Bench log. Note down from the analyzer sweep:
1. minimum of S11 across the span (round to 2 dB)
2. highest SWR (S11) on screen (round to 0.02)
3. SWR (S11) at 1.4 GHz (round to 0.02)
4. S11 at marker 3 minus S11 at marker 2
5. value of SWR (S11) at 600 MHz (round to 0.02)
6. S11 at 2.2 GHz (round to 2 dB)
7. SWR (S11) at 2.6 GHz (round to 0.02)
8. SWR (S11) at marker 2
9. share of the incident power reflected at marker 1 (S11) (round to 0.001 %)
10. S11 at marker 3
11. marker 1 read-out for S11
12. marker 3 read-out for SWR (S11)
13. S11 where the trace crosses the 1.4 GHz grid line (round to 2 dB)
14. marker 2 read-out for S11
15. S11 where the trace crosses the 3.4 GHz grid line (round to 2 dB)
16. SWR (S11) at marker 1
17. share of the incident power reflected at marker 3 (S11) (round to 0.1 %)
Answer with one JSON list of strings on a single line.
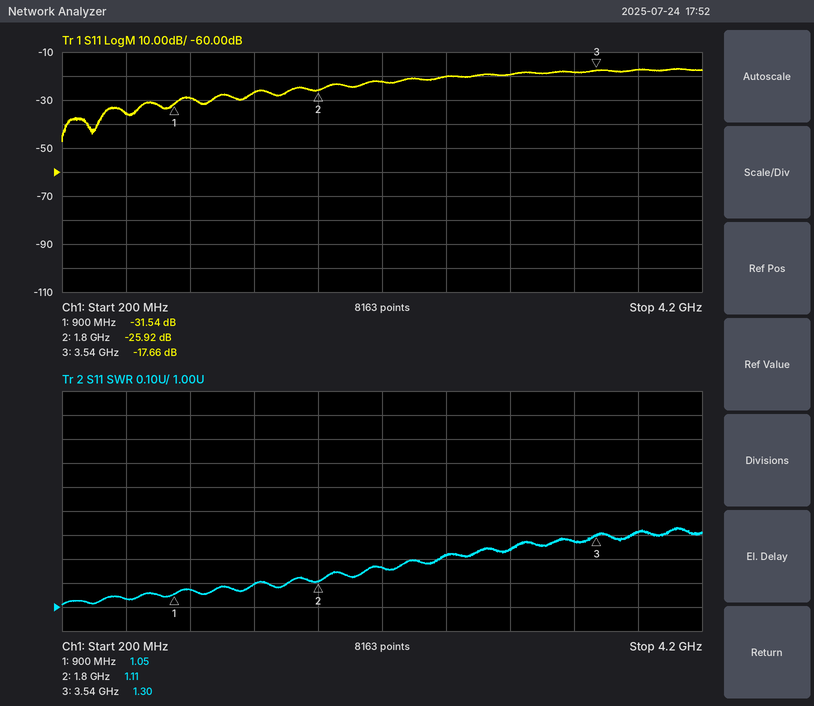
["-48 dB", "1.34", "1.10", "8.26 dB", "1.04", "-22 dB", "1.22", "1.11", "0.070 %", "-17.66 dB", "-31.54 dB", "1.30", "-26 dB", "-25.92 dB", "-18 dB", "1.05", "1.7 %"]
